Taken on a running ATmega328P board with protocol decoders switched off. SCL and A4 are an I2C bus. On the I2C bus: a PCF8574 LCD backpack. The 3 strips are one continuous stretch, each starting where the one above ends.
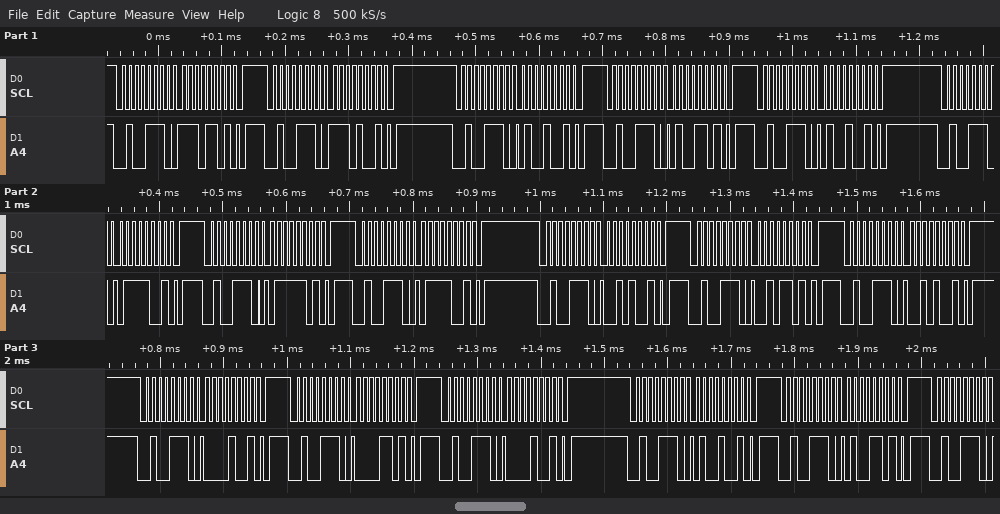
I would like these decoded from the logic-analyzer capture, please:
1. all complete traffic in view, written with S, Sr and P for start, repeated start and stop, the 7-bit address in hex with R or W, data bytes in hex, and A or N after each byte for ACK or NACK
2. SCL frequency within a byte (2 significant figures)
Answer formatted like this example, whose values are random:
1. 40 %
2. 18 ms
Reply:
1. S 27W A ED A P S 27W A E9 A P S 27W A 49 A P S 27W A 4D A P S 27W A 49 A P S 27W A 79 A P S 27W A 7D A P S 27W A 79 A P S 27W A 29 A P S 27W A 2D A P S 27W A 29 A P S 27W A 09 A P S 27W A 0D A P S 27W A 09 A P S 27W A 49 A P S 27W A 4D A P S 27W A
2. 100 kHz
